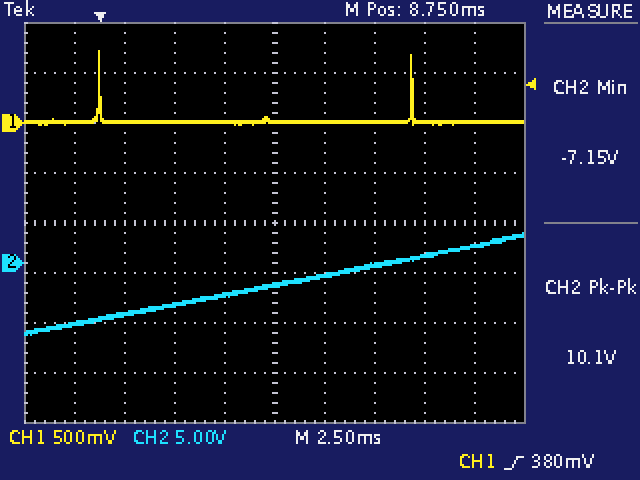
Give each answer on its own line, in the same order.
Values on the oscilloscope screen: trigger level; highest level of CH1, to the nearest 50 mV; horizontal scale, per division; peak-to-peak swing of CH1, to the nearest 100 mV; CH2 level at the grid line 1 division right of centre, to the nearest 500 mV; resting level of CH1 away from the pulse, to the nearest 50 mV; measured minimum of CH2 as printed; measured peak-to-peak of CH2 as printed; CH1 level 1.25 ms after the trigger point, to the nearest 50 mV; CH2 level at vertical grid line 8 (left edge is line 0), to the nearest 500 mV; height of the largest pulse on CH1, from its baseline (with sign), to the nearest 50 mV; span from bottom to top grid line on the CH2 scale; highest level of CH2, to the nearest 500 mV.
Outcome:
380 mV
700 mV
2.5 ms
700 mV
-1.0 V
0 mV
-7.15 V
10.1 V
0 mV
1.0 V
+700 mV
40 V
3.0 V
